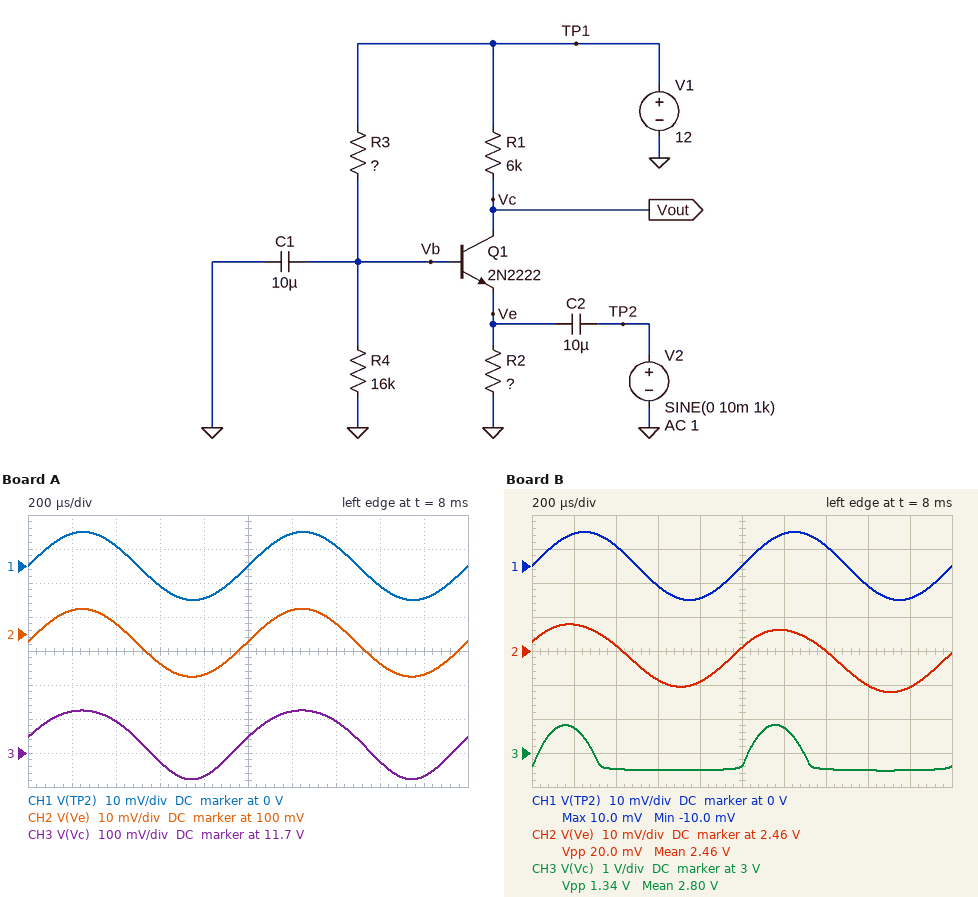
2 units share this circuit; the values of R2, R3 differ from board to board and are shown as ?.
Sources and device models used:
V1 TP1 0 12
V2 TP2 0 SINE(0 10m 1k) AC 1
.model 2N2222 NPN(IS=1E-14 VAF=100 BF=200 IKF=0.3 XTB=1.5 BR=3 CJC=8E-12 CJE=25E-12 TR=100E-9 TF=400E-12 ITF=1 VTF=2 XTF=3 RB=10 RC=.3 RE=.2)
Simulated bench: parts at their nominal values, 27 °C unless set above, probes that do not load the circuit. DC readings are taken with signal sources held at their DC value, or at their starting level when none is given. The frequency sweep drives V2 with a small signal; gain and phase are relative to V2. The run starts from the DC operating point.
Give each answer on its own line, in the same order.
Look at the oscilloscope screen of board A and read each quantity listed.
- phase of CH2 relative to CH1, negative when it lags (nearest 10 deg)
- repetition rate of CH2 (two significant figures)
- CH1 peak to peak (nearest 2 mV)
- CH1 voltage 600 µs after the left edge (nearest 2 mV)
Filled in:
0 deg
1.0 kHz
20 mV
-6 mV
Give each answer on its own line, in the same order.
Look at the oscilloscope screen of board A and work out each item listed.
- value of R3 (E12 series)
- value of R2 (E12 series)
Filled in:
270 kΩ
2.2 kΩ
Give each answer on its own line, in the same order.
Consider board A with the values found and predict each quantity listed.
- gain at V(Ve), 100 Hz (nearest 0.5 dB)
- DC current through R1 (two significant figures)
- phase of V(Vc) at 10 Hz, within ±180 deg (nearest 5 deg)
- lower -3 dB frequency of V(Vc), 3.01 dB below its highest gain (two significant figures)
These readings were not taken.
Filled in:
-0.5 dB
44 µA
75 deg
34 Hz
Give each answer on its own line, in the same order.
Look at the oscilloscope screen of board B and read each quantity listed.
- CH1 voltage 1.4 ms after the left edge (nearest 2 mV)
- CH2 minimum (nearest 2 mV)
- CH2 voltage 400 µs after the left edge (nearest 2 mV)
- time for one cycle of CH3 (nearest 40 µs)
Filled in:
6 mV
2.448 V
2.462 V
1.00 ms
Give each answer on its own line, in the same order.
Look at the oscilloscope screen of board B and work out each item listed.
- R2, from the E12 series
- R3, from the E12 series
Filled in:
1.5 kΩ
33 kΩ
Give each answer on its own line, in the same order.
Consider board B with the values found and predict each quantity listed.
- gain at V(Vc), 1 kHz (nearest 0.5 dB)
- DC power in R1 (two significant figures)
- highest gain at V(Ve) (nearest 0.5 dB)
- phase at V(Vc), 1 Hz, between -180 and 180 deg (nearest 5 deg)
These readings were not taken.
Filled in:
15.0 dB
15 mW
0 dB
85 deg
